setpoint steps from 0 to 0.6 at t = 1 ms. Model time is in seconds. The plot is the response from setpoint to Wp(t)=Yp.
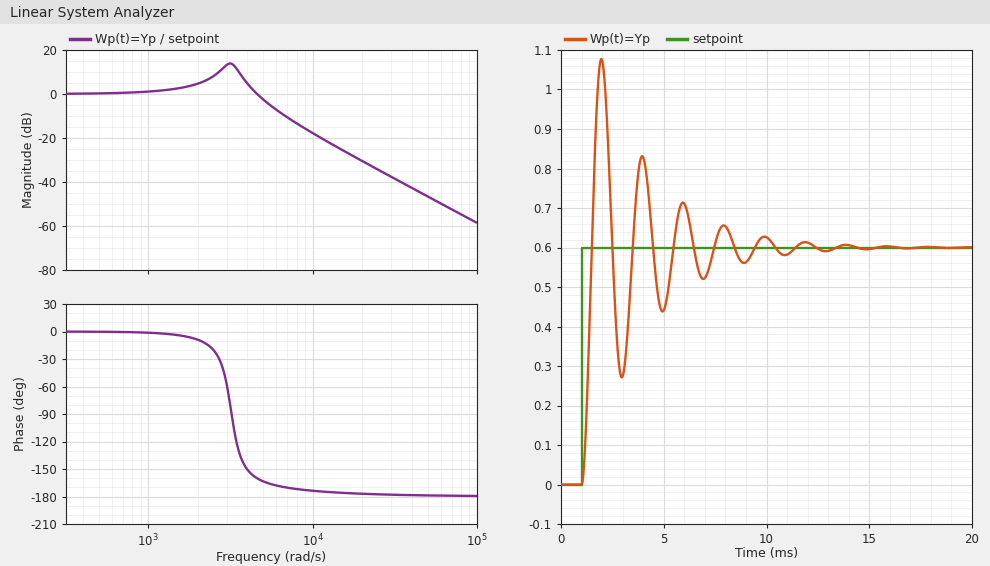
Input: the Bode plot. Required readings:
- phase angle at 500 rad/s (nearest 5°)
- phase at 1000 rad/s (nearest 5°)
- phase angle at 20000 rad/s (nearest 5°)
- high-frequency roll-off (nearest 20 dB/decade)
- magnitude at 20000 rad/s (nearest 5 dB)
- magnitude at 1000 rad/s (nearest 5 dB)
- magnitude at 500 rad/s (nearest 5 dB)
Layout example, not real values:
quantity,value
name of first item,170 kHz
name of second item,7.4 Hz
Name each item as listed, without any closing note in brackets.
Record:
quantity,value
phase angle at 500 rad/s,0°
phase at 1000 rad/s,0°
phase angle at 20000 rad/s,-175°
high-frequency roll-off,-40 dB/decade
magnitude at 20000 rad/s,-30 dB
magnitude at 1000 rad/s,0 dB
magnitude at 500 rad/s,0 dB
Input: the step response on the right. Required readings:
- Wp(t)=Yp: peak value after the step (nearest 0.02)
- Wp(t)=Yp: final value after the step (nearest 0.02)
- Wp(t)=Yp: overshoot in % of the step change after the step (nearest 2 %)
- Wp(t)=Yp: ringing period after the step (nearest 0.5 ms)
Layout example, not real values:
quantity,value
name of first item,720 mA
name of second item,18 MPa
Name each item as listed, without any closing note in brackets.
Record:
quantity,value
Wp(t)=Yp: peak value after the step,1.08
Wp(t)=Yp: final value after the step,0.60
Wp(t)=Yp: overshoot in % of the step change after the step,80 %
Wp(t)=Yp: ringing period after the step,2.0 ms
